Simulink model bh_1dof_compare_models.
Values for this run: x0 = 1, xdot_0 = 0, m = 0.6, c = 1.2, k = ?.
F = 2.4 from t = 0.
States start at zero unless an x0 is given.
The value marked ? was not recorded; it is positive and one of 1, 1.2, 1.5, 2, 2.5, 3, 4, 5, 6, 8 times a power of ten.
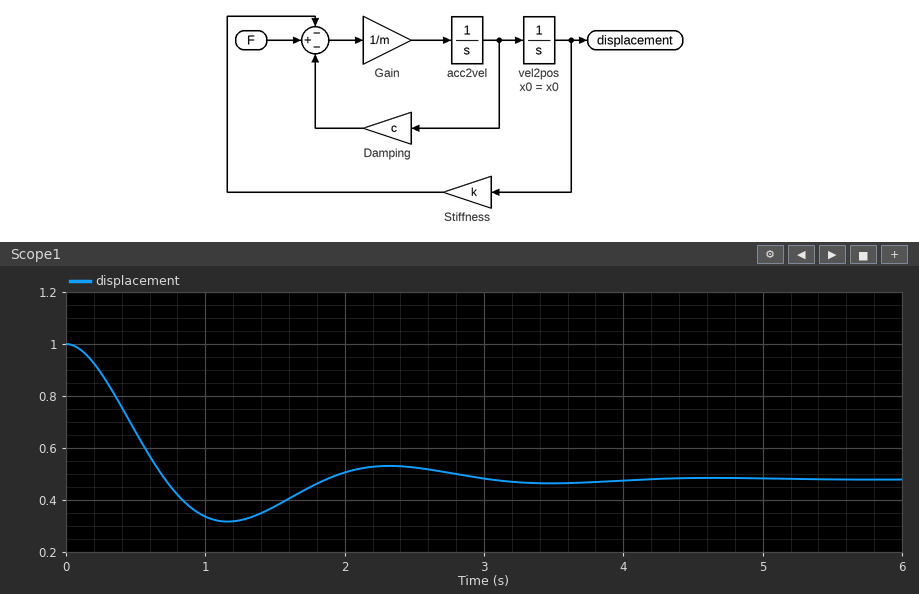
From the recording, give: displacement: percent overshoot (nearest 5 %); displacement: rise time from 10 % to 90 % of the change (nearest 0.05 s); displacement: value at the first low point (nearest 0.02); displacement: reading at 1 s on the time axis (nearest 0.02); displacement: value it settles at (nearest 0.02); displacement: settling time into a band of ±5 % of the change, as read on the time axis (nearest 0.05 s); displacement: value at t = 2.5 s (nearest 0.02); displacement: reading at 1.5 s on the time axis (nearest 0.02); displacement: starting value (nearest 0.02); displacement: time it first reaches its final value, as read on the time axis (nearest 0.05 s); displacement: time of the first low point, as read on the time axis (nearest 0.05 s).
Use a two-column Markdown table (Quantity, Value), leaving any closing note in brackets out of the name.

| Quantity | Value |
|---|---|
| displacement: percent overshoot | 30 % |
| displacement: rise time from 10 % to 90 % of the change | 0.50 s |
| displacement: value at the first low point | 0.32 |
| displacement: reading at 1 s on the time axis | 0.34 |
| displacement: value it settles at | 0.48 |
| displacement: settling time into a band of ±5 % of the change, as read on the time axis | 2.75 s |
| displacement: value at t = 2.5 s | 0.52 |
| displacement: reading at 1.5 s on the time axis | 0.38 |
| displacement: starting value | 1.00 |
| displacement: time it first reaches its final value, as read on the time axis | 0.70 s |
| displacement: time of the first low point, as read on the time axis | 1.15 s |
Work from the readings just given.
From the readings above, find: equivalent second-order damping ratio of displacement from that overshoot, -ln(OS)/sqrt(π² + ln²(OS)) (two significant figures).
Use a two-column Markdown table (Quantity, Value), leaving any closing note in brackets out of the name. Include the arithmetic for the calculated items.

| Quantity | Value |
|---|---|
| equivalent second-order damping ratio of displacement from that overshoot, -ln(OS)/sqrt(π² + ln²(OS)) | ln(0.3) = -1.204; 1.204 / sqrt(9.870 + 1.450) = 0.36 |
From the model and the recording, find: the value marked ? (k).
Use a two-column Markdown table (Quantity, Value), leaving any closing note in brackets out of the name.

| Quantity | Value |
|---|---|
| the value marked ? | 5 |
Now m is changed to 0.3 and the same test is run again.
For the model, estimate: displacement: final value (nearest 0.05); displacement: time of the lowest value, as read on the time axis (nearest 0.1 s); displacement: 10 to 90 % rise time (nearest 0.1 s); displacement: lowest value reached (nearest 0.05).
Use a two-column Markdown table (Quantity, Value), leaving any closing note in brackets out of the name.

| Quantity | Value |
|---|---|
| displacement: final value | 0.50 |
| displacement: time of the lowest value, as read on the time axis | 0.9 s |
| displacement: 10 to 90 % rise time | 0.4 s |
| displacement: lowest value reached | 0.40 |
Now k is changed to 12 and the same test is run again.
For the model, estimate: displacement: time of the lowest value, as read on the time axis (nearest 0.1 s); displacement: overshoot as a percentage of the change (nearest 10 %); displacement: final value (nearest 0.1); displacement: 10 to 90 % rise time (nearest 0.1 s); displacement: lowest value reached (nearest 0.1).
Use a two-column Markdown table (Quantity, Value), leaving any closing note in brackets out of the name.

| Quantity | Value |
|---|---|
| displacement: time of the lowest value, as read on the time axis | 0.7 s |
| displacement: overshoot as a percentage of the change | 50 % |
| displacement: final value | 0.2 |
| displacement: 10 to 90 % rise time | 0.3 s |
| displacement: lowest value reached | -0.2 |
